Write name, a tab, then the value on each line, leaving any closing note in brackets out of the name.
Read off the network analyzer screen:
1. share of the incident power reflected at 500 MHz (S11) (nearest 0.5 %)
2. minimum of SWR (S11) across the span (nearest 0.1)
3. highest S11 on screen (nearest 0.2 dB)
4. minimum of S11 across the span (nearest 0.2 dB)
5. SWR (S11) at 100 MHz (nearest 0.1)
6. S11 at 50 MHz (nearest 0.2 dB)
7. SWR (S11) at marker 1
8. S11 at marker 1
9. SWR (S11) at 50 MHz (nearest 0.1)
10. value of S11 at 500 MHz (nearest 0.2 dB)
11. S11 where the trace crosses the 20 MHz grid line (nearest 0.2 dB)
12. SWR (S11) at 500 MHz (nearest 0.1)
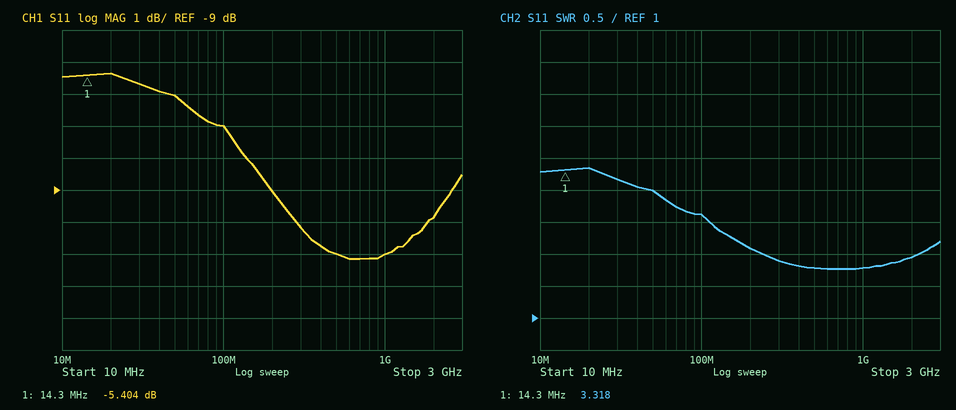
share of the incident power reflected at 500 MHz (S11)	8.0 %
minimum of SWR (S11) across the span	1.8
highest S11 on screen	-5.4 dB
minimum of S11 across the span	-11.2 dB
SWR (S11) at 100 MHz	2.6
S11 at 50 MHz	-6.0 dB
SWR (S11) at marker 1	3.318
S11 at marker 1	-5.404 dB
SWR (S11) at 50 MHz	3.0
value of S11 at 500 MHz	-11.0 dB
S11 where the trace crosses the 20 MHz grid line	-5.4 dB
SWR (S11) at 500 MHz	1.8
